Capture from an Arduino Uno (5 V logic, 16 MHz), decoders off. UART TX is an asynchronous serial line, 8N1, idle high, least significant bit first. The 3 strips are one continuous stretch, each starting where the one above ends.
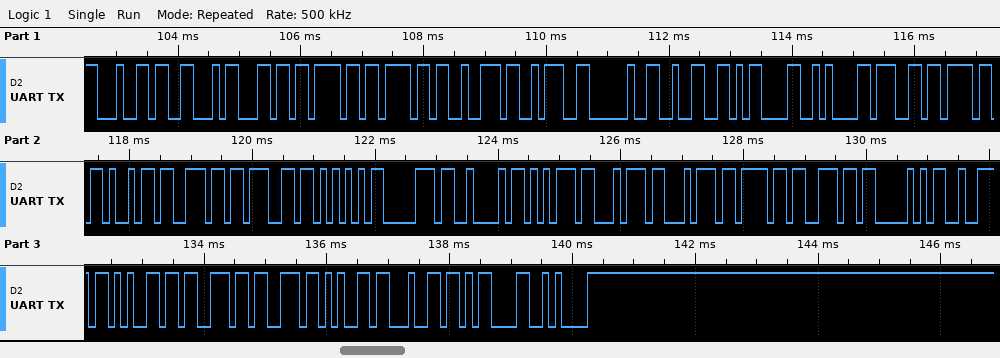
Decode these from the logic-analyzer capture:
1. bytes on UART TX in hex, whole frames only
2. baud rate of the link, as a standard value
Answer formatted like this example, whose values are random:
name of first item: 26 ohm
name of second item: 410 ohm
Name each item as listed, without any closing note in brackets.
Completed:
bytes on UART TX in hex, whole frames only: 64 46 6C 6F 6F 72 3A 20 32 0D 0A 67 6F 69 6E 67 55 70 42 75 74 74 6F 6E 50 72 65 73 73 65 64 0D 0A
baud rate of the link, as a standard value: 9600 baud
